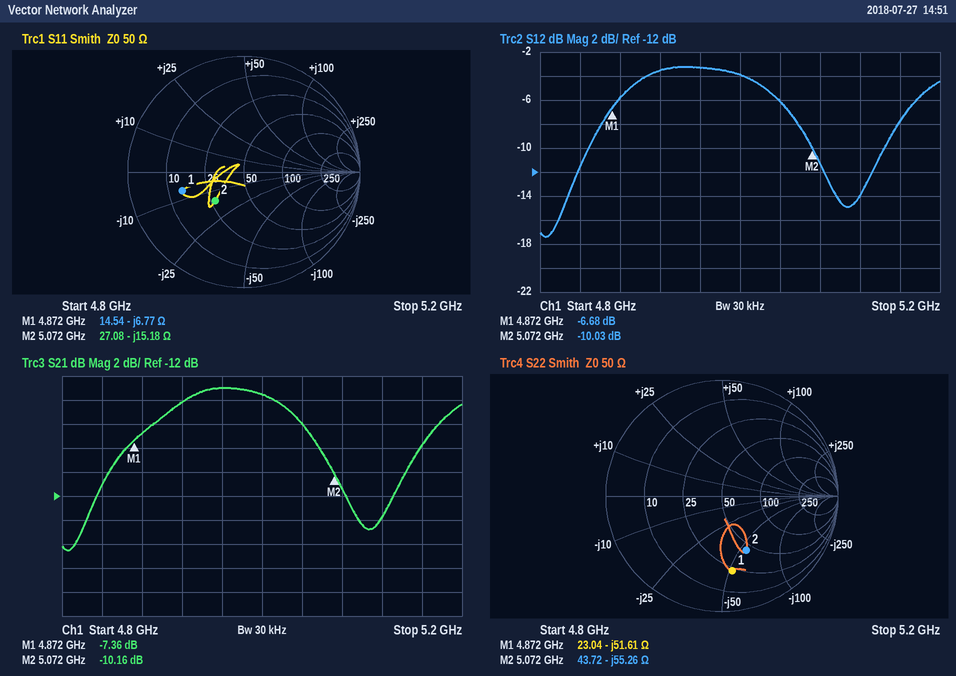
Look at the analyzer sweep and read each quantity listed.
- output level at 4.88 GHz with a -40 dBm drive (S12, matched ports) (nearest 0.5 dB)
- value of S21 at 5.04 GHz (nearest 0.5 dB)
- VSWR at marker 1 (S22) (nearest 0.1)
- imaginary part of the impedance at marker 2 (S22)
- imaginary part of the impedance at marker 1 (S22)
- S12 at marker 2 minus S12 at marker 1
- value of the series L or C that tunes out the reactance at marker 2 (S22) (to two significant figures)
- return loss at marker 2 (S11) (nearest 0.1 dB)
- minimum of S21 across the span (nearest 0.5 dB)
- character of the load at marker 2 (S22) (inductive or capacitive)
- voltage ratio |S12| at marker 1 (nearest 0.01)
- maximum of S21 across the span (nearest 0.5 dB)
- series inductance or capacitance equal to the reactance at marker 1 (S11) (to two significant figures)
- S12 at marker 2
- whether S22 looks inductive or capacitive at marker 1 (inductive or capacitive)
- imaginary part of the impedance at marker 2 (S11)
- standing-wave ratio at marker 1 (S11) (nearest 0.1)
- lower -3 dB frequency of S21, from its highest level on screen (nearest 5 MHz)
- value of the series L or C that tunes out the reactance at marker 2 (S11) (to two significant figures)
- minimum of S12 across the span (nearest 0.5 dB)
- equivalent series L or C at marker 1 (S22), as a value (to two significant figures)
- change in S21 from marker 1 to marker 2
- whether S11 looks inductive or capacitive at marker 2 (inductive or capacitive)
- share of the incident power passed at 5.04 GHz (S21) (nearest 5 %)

-46.0 dBm
-6.0 dB
4.7
-55.26 Ω
-51.61 Ω
-3.35 dB
1.7 nH
9.1 dB
-16.5 dB
capacitive
0.46
-3.0 dB
4.8 pF
-10.03 dB
capacitive
-15.18 Ω
3.5
4.890 GHz
480 pH
-17.5 dB
630 fF
-2.80 dB
capacitive
25 %
